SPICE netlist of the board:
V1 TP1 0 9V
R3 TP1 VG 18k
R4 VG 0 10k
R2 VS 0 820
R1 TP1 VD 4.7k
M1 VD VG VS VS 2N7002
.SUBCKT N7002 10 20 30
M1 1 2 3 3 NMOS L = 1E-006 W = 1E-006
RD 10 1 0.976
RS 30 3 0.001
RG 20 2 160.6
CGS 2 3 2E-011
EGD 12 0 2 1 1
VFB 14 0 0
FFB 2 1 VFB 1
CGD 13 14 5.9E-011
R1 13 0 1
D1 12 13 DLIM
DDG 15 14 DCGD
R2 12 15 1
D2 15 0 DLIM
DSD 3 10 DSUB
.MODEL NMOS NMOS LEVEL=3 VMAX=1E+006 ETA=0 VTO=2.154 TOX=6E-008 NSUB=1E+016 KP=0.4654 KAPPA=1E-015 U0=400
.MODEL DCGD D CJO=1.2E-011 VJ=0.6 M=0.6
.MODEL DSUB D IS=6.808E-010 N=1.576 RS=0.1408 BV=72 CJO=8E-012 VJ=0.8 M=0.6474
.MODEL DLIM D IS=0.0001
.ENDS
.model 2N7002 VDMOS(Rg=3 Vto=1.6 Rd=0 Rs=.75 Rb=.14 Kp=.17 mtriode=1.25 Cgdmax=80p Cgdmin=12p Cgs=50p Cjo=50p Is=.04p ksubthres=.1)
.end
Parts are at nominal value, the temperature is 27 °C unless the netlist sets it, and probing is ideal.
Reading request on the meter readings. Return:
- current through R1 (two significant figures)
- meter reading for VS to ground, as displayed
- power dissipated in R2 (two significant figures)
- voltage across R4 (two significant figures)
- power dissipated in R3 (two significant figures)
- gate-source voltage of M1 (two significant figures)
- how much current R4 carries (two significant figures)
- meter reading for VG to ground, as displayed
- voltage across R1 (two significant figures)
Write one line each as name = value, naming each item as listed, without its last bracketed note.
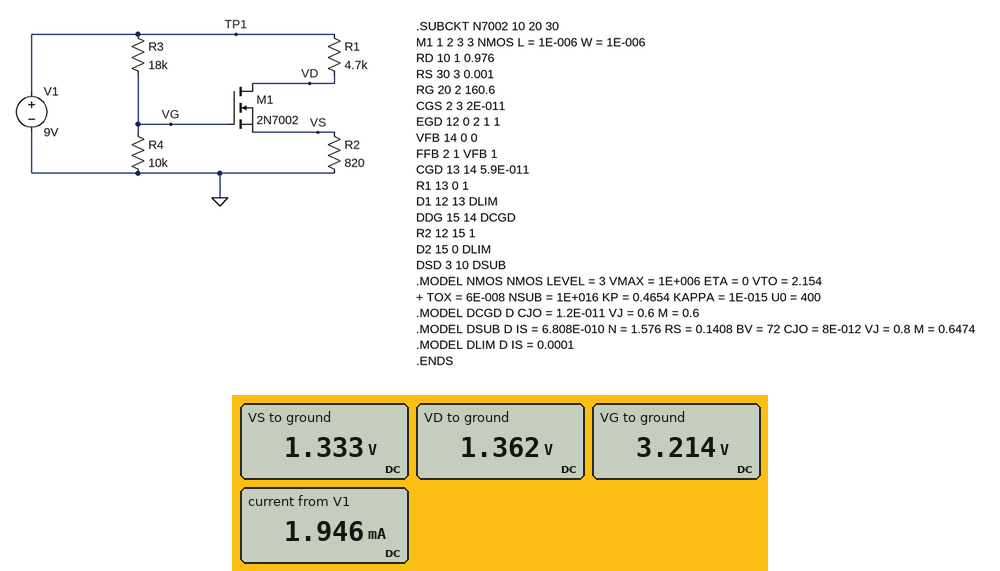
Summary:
current through R1 = 1.6 mA
meter reading for VS to ground, as displayed = 1.333 V
power dissipated in R2 = 2.2 mW
voltage across R4 = 3.2 V
power dissipated in R3 = 1.9 mW
gate-source voltage of M1 = 1.9 V
how much current R4 carries = 320 µA
meter reading for VG to ground, as displayed = 3.214 V
voltage across R1 = 7.6 V
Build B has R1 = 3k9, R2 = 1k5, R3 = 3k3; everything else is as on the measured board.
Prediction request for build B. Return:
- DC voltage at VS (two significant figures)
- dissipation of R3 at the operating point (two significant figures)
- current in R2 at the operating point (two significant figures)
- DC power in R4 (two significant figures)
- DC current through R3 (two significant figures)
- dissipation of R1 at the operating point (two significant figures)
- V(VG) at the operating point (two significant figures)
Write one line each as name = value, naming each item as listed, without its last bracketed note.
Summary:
DC voltage at VS = 2.5 V
dissipation of R3 at the operating point = 1.5 mW
current in R2 at the operating point = 1.7 mA
DC power in R4 = 4.6 mW
DC current through R3 = 680 µA
dissipation of R1 at the operating point = 11 mW
V(VG) at the operating point = 6.8 V
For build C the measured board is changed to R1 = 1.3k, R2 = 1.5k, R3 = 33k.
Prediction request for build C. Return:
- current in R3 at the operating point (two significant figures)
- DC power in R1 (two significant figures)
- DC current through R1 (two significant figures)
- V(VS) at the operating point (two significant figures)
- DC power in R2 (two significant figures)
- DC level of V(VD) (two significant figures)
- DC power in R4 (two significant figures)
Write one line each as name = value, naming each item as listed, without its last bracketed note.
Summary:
current in R3 at the operating point = 210 µA
DC power in R1 = 150 µW
DC current through R1 = 340 µA
V(VS) at the operating point = 510 mV
DC power in R2 = 170 µW
DC level of V(VD) = 8.6 V
DC power in R4 = 440 µW
